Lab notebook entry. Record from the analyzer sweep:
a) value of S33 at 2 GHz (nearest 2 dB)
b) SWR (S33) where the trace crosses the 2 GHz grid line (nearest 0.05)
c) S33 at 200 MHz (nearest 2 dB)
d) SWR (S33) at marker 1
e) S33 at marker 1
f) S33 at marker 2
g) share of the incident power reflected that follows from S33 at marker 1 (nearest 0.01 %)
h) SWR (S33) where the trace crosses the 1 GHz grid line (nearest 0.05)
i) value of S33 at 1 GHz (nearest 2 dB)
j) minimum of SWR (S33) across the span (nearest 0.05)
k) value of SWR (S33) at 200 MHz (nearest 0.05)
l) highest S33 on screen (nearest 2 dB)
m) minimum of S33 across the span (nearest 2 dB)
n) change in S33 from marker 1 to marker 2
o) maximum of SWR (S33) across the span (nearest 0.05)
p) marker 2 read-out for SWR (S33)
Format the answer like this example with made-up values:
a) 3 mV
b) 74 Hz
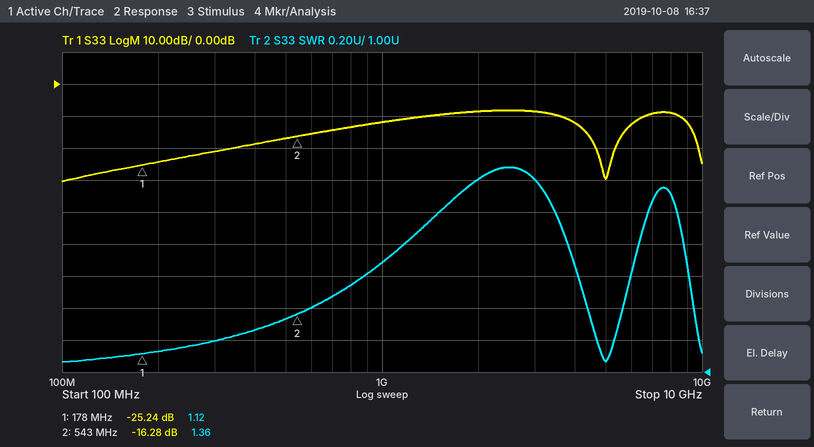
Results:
a) -8 dB
b) 2.20
c) -24 dB
d) 1.12
e) -25.24 dB
f) -16.28 dB
g) 0.30 %
h) 1.70
i) -12 dB
j) 1.05
k) 1.15
l) -8 dB
m) -30 dB
n) 8.96 dB
o) 2.30
p) 1.36
